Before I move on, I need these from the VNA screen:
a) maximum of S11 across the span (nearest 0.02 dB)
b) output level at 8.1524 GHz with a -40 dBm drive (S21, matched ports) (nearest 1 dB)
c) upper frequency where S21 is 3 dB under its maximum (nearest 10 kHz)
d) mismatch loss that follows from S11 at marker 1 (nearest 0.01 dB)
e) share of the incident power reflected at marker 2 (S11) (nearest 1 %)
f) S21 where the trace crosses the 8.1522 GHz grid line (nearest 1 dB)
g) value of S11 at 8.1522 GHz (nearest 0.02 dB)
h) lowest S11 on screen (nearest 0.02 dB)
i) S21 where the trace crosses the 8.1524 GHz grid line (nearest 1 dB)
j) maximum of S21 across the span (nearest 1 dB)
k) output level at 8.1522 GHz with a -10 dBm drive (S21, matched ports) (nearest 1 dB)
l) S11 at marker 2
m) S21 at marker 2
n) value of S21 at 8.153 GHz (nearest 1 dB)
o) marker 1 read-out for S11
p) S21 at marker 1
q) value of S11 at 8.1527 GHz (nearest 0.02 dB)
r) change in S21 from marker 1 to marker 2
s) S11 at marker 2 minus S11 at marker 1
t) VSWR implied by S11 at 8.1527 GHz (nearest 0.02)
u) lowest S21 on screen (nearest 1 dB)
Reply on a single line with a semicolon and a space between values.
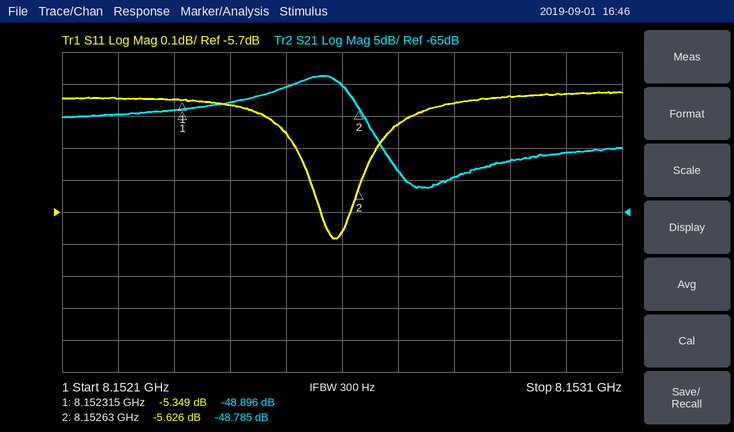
-5.32 dB; -88 dBm; 8.15261 GHz; 1.50 dB; 27 %; -50 dB; -5.34 dB; -5.78 dB; -48 dB; -44 dB; -60 dBm; -5.626 dB; -48.785 dB; -56 dB; -5.349 dB; -48.896 dB; -5.42 dB; 0.111 dB; -0.277 dB; 3.30; -61 dB
